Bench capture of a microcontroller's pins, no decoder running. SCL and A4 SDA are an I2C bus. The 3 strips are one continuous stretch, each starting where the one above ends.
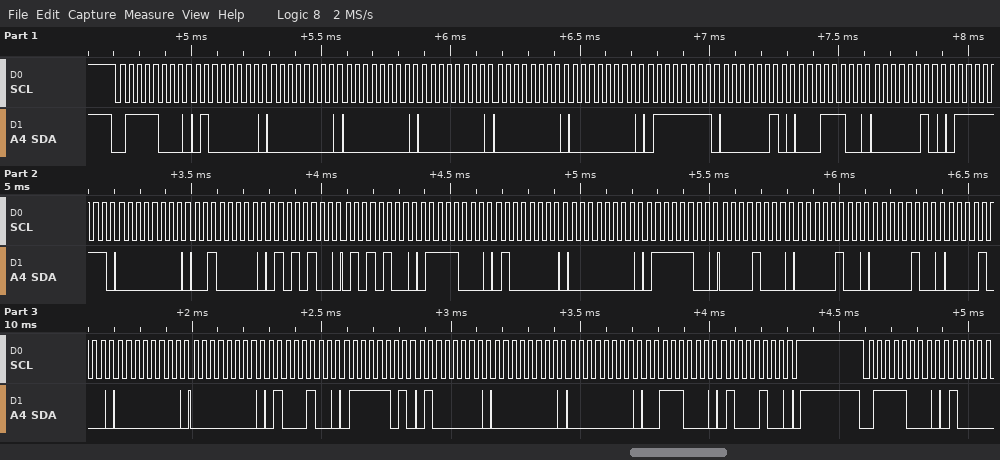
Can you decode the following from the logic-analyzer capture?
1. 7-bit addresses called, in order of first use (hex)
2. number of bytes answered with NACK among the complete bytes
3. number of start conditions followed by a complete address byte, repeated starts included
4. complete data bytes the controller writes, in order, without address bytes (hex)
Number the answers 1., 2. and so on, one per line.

1. 0x3C
2. 0
3. 2
4. 40 00 00 00 00 00 7F 02 1C 02 7F 00 20 54 54 78 40 00 7C 08 04 04 08 00 00 44 7D 40 00 00 38 44
